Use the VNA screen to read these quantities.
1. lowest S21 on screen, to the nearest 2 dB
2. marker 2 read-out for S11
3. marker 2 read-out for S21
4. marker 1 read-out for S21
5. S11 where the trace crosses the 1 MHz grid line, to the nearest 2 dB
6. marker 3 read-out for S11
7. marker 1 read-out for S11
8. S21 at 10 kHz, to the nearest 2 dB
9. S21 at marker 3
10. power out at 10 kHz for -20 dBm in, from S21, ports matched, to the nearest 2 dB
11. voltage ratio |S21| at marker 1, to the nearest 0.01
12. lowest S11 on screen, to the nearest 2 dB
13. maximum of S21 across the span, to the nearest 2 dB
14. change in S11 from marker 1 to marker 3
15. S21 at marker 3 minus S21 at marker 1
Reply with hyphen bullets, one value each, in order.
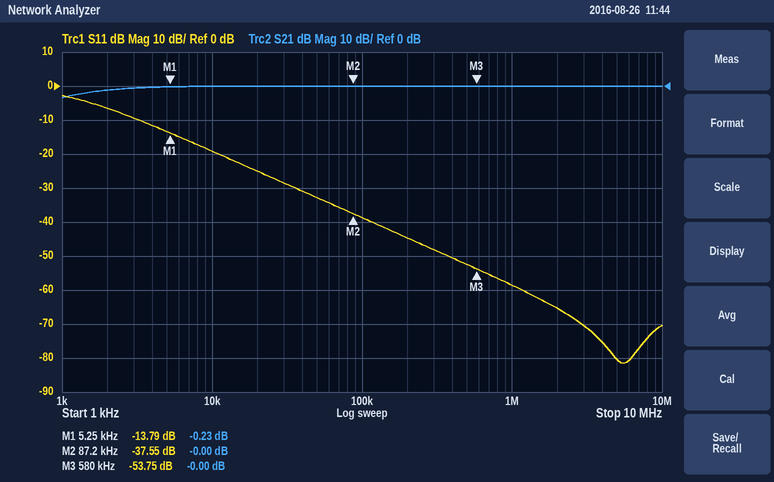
- -4 dB
- -37.55 dB
- -0.00 dB
- -0.23 dB
- -58 dB
- -53.75 dB
- -13.79 dB
- 0 dB
- -0.00 dB
- -20 dBm
- 0.97
- -82 dB
- 0 dB
- -39.96 dB
- 0.23 dB
